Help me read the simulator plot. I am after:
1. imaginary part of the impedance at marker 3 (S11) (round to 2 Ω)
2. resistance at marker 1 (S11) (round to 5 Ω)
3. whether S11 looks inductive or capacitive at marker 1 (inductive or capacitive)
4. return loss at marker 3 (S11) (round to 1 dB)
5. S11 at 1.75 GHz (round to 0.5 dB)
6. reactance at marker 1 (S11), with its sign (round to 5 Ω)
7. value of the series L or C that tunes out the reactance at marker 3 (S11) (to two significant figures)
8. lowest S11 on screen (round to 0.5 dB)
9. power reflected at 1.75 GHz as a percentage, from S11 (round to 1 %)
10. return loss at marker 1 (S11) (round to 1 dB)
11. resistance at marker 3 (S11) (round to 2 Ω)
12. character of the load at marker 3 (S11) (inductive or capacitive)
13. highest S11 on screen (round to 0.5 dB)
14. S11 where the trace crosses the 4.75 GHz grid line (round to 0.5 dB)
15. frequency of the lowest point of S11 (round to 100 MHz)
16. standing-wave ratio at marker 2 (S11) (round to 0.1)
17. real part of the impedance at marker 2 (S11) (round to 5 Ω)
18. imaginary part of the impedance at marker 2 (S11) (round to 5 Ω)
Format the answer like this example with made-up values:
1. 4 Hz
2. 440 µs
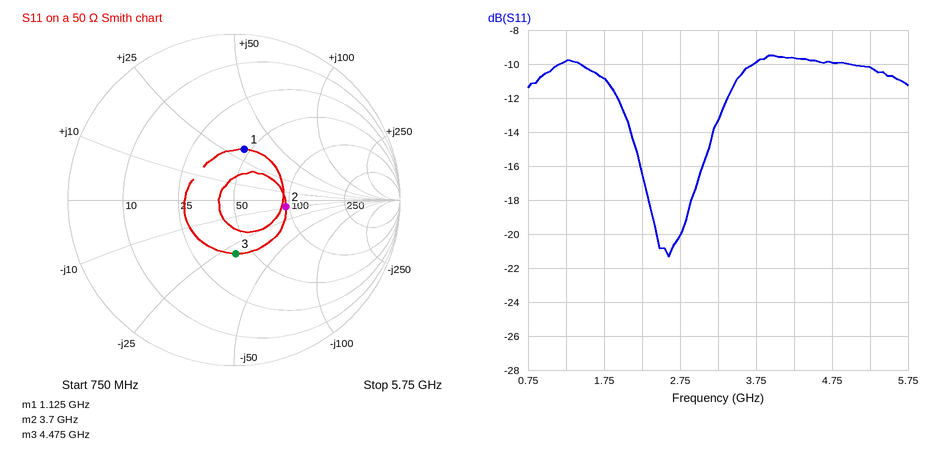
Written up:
1. -30 Ω
2. 45 Ω
3. inductive
4. 10 dB
5. -11.0 dB
6. +30 Ω
7. 1.1 nH
8. -21.5 dB
9. 8 %
10. 10 dB
11. 42 Ω
12. capacitive
13. -9.5 dB
14. -10.0 dB
15. 2.6 GHz
16. 1.9
17. 95 Ω
18. -10 Ω
